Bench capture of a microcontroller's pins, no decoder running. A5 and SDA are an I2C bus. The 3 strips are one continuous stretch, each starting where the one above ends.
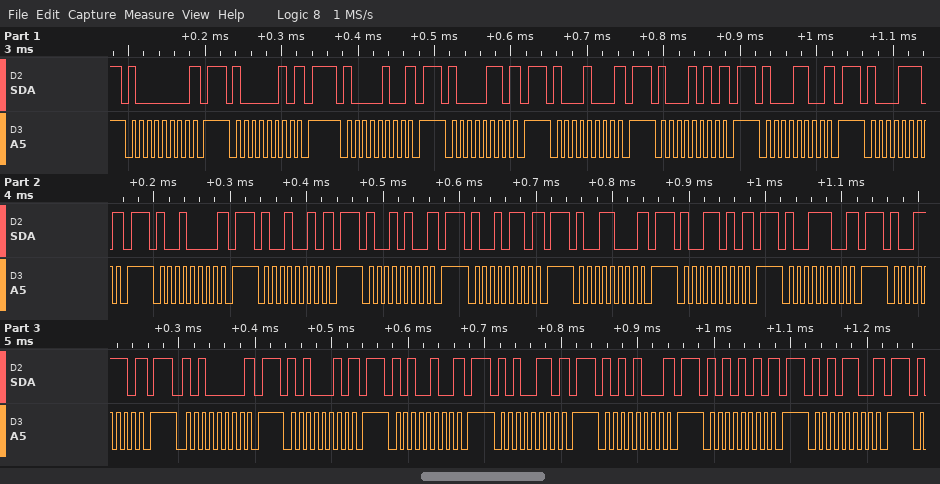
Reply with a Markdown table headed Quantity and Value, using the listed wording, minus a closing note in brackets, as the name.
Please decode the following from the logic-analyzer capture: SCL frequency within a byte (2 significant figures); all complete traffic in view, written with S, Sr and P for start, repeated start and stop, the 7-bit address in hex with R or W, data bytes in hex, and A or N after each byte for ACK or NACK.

| Quantity | Value |
|---|---|
| SCL frequency within a byte | 100 kHz |
| all complete traffic in view, written with S, Sr and P for start, repeated start and stop, the 7-bit address in hex with R or W, data bytes in hex, and A or N after each byte for ACK or NACK | S 40W N P S 41W N P S 42W N P S 43W N P S 44W N P S 45W N P S 46W N P S 47W N P S 48W N P S 49W N P S 4AW N P S 4BW N P S 4CW N P S 4DW N P S 4EW N P S 4FW N P S 50W N P S 51W N P S 52W N P S 53W N P S 54W N P S 55W N P S 56W N P |
